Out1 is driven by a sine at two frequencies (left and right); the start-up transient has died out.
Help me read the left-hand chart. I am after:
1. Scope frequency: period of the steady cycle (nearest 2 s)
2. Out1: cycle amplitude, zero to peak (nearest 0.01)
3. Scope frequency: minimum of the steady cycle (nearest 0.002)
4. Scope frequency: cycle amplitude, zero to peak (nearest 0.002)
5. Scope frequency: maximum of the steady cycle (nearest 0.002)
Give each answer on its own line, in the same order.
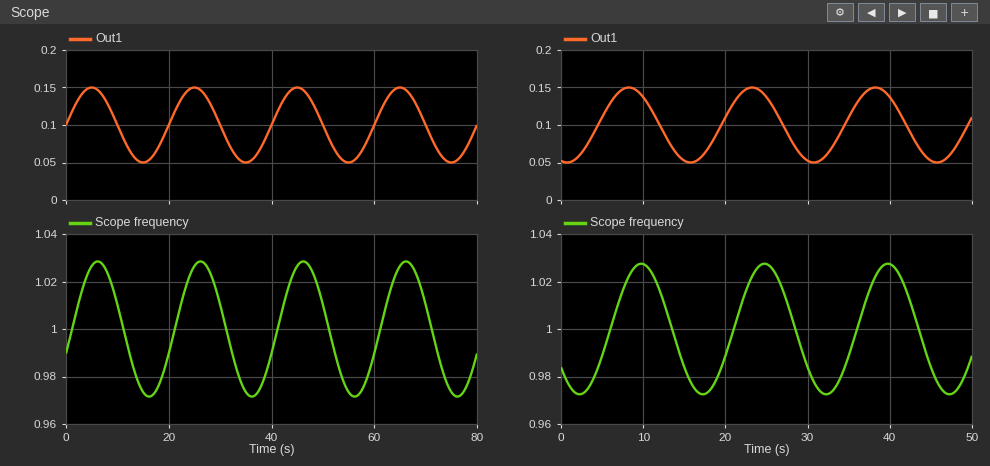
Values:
20 s
0.05
0.972
0.028
1.028
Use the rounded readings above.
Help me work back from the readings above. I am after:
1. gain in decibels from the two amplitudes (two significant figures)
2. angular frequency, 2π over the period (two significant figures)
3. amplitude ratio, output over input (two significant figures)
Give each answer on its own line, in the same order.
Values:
-5.0 dB
0.31 rad/s
0.56
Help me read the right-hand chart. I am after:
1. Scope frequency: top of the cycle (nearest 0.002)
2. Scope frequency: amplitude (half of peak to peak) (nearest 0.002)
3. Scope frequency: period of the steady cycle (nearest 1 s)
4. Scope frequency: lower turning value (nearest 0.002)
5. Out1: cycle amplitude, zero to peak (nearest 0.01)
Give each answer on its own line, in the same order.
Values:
1.028
0.028
15 s
0.972
0.05
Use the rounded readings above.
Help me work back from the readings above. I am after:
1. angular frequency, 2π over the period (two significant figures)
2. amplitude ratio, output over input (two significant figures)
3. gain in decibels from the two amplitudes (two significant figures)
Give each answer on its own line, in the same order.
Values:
0.42 rad/s
0.56
-5.0 dB
